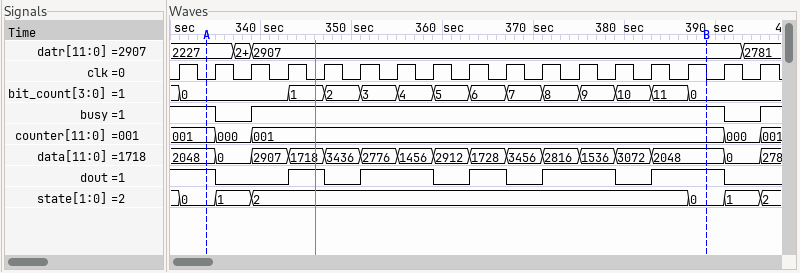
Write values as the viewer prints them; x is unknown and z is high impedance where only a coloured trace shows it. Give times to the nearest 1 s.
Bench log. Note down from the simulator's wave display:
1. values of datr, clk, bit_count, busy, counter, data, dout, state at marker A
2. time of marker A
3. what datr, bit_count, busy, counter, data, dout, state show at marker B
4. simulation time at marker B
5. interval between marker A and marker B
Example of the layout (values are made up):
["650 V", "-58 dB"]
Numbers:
["datr=2227, clk=0, bit_count=0, busy=1, counter=001, data=2048, dout=1, state=0", "334 s", "datr=2907, bit_count=0, busy=1, counter=001, data=2048, dout=1, state=0", "389 s", "55 s"]
